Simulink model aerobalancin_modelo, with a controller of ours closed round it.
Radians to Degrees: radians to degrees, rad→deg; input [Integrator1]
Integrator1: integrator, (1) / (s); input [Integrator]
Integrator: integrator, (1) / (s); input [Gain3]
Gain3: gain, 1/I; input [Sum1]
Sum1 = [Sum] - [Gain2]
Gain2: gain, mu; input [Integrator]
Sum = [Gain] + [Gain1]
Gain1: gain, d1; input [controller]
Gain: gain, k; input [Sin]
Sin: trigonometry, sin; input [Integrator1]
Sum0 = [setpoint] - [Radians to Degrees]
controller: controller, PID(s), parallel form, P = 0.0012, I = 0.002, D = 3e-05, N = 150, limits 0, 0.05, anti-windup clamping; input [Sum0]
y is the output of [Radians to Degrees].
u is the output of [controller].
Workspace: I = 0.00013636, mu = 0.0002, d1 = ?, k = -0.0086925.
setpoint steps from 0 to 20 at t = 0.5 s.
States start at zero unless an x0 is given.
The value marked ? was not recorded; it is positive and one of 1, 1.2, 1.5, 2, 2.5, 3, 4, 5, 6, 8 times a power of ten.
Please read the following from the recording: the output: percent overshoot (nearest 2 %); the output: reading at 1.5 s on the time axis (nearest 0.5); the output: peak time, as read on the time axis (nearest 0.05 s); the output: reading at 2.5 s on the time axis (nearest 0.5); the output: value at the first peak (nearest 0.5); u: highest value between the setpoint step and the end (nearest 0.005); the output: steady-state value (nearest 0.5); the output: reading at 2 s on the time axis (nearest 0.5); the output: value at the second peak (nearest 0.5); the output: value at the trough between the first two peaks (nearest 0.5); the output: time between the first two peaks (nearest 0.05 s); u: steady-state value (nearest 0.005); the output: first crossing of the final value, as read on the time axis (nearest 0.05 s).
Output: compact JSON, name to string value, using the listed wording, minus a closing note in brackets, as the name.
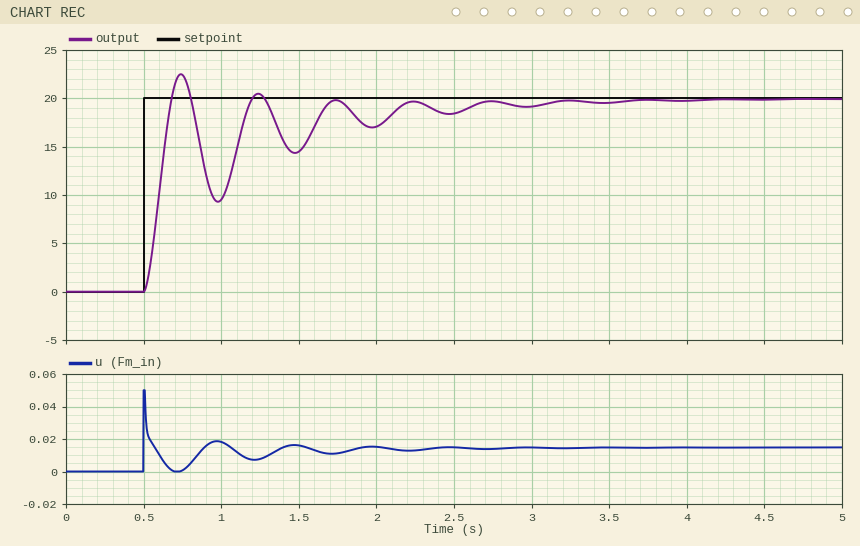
{"the output: percent overshoot": "12 %", "the output: reading at 1.5 s on the time axis": "14.5", "the output: peak time, as read on the time axis": "0.75 s", "the output: reading at 2.5 s on the time axis": "18.5", "the output: value at the first peak": "22.5", "u: highest value between the setpoint step and the end": "0.050", "the output: steady-state value": "20.0", "the output: reading at 2 s on the time axis": "17.0", "the output: value at the second peak": "20.5", "the output: value at the trough between the first two peaks": "9.5", "the output: time between the first two peaks": "0.50 s", "u: steady-state value": "0.015", "the output: first crossing of the final value, as read on the time axis": "0.70 s"}
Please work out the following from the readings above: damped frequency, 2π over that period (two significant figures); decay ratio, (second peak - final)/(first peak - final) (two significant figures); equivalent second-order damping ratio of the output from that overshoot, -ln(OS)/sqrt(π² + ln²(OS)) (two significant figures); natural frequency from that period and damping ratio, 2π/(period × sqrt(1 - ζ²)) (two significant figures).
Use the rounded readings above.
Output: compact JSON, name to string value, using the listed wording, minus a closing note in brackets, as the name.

{"damped frequency, 2π over that period": "13 rad/s", "decay ratio, (second peak - final)/(first peak - final)": "0.20", "equivalent second-order damping ratio of the output from that overshoot, -ln(OS)/sqrt(π² + ln²(OS))": "0.56", "natural frequency from that period and damping ratio, 2π/(period × sqrt(1 - ζ²))": "15 rad/s"}
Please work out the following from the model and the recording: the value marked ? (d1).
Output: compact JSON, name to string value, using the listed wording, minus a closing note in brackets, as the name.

{"the value marked ?": "0.2"}
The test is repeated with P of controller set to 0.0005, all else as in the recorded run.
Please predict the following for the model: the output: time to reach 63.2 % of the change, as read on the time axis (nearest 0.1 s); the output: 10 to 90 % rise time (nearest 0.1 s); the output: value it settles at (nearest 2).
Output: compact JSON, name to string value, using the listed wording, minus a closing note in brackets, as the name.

{"the output: time to reach 63.2 % of the change, as read on the time axis": "0.7 s", "the output: 10 to 90 % rise time": "0.8 s", "the output: value it settles at": "20"}
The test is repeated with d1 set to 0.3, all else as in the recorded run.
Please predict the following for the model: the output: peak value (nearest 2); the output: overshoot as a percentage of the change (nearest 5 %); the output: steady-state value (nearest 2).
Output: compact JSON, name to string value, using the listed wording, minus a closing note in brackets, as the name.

{"the output: peak value": "26", "the output: overshoot as a percentage of the change": "30 %", "the output: steady-state value": "20"}
